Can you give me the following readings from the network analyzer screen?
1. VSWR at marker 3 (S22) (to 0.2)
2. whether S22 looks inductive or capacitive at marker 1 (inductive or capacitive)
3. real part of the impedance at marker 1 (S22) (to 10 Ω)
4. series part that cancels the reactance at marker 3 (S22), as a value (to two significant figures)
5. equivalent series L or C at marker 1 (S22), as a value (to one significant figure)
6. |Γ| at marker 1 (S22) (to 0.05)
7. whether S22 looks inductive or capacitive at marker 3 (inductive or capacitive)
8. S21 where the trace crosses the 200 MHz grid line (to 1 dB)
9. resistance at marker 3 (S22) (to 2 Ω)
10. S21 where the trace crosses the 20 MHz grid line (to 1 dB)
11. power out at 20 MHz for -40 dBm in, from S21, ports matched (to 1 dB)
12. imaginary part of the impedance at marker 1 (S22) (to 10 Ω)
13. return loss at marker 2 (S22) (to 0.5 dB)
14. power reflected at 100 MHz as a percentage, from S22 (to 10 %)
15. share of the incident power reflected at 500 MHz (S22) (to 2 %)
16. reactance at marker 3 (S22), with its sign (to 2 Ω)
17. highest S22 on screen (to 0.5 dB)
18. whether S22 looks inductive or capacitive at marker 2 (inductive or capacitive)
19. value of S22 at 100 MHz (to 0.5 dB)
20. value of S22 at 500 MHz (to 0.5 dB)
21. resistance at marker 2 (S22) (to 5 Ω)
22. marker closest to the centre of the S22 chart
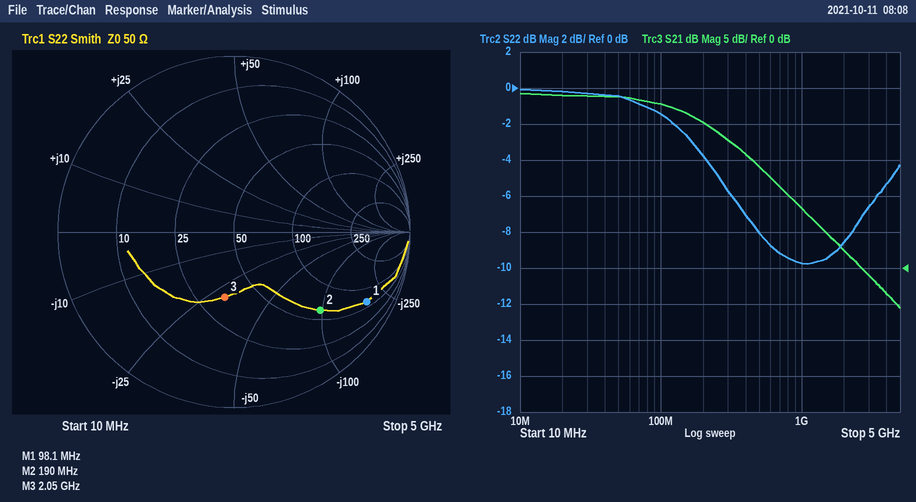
2.2
capacitive
60 Ω
2.3 nH
9 pF
0.85
capacitive
20 dB
34 Ω
24 dB
-16 dBm
-180 Ω
3.5 dB
70 %
16 %
-30 Ω
0.0 dB
capacitive
-1.5 dB
-8.0 dB
60 Ω
marker 3
